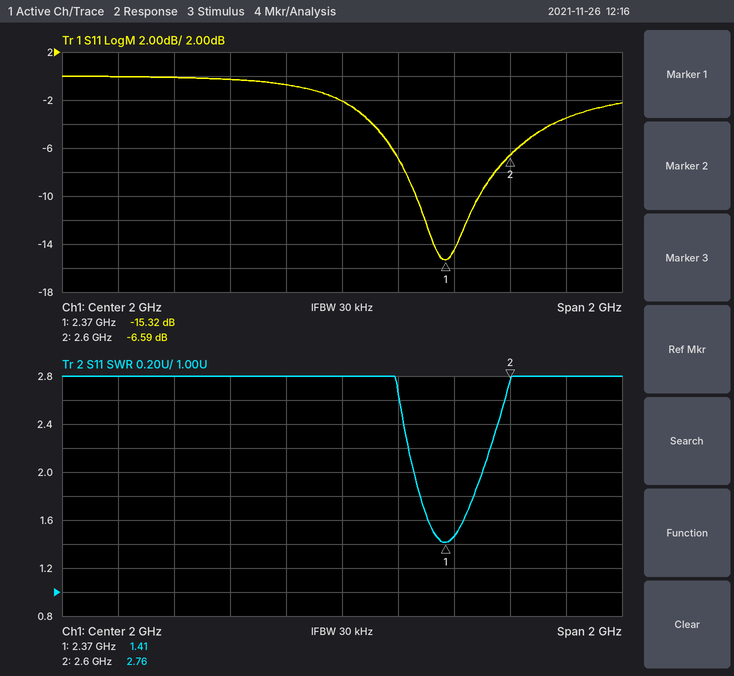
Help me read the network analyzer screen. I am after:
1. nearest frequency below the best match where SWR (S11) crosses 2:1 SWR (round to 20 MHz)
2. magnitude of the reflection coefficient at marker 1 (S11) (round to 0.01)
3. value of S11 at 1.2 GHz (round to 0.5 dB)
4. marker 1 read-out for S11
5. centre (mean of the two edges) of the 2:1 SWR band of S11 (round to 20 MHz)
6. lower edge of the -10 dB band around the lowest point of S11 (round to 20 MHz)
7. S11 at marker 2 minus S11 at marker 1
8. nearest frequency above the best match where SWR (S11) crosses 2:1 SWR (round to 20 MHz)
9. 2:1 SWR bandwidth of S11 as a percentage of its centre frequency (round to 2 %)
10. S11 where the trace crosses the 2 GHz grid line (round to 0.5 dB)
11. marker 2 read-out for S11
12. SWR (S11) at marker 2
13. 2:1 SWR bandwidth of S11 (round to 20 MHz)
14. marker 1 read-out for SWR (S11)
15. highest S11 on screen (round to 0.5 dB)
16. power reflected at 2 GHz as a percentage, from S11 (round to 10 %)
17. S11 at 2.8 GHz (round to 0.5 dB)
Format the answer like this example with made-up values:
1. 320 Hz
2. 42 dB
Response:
1. 2.26 GHz
2. 0.17
3. 0.0 dB
4. -15.32 dB
5. 2.38 GHz
6. 2.26 GHz
7. 8.73 dB
8. 2.50 GHz
9. 10 %
10. -2.0 dB
11. -6.59 dB
12. 2.76
13. 240 MHz
14. 1.41
15. 0.0 dB
16. 60 %
17. -3.5 dB
